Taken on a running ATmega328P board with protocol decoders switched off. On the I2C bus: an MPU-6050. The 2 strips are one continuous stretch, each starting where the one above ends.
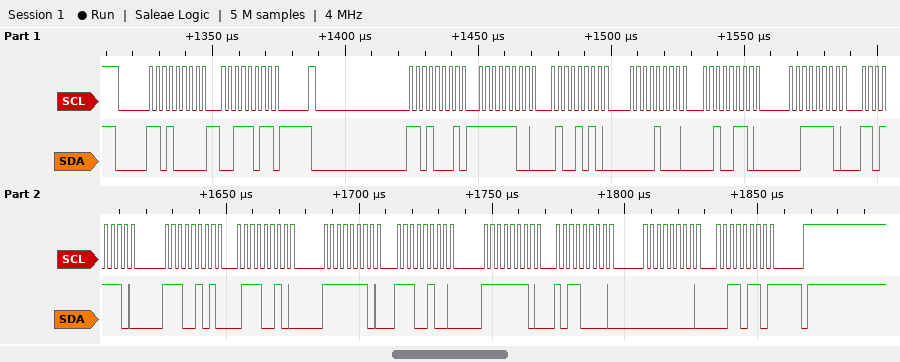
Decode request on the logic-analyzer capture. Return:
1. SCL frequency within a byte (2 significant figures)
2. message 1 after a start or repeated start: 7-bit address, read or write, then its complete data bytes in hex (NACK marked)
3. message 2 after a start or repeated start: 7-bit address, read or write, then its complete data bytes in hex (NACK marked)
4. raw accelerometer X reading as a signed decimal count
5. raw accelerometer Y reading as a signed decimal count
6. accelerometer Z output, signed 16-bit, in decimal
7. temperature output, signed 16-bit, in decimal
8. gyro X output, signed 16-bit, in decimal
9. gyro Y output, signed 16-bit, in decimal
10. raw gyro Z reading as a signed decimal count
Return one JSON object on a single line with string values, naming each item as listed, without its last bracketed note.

{"SCL frequency within a byte": "400 kHz", "message 1 after a start or repeated start: 7-bit address, read or write, then its complete data bytes in hex": "0x68 write: 3B", "message 2 after a start or repeated start: 7-bit address, read or write, then its complete data bytes in hex": "0x68 read: FC 4A 08 26 3E DE E5 72 FE E4 FE B0 00 36 NACK", "raw accelerometer X reading as a signed decimal count": "-950", "raw accelerometer Y reading as a signed decimal count": "2086", "accelerometer Z output, signed 16-bit, in decimal": "16094", "temperature output, signed 16-bit, in decimal": "-6798", "gyro X output, signed 16-bit, in decimal": "-284", "gyro Y output, signed 16-bit, in decimal": "-336", "raw gyro Z reading as a signed decimal count": "54"}
